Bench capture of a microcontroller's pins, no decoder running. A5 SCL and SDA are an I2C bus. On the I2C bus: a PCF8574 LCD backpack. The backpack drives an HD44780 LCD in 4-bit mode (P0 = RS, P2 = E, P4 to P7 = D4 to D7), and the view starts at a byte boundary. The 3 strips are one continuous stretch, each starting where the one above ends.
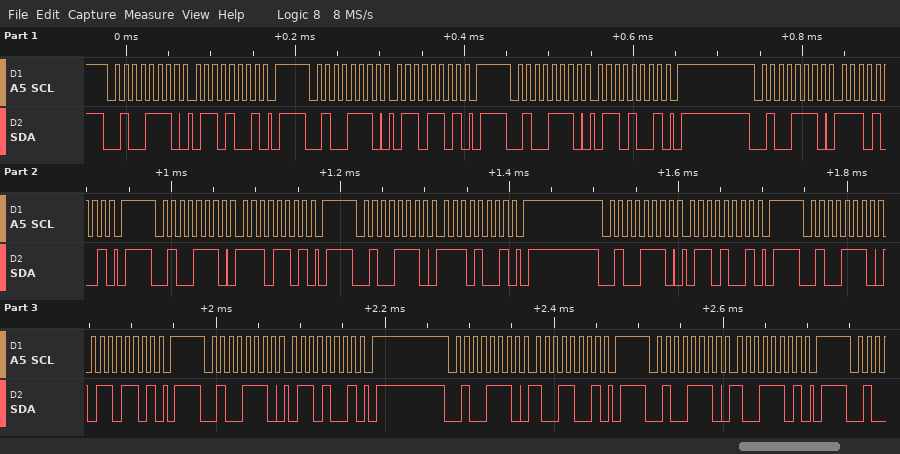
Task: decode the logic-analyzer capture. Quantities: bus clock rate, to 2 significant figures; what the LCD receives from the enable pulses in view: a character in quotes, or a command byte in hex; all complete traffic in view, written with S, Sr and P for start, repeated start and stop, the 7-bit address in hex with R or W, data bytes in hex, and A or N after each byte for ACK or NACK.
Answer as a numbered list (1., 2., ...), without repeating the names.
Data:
1. 100 kHz
2. 'n'
3. S 27W A 69 A P S 27W A 6D A P S 27W A 69 A P S 27W A E9 A P S 27W A ED A P S 27W A E9 A P S 27W A 69 A P S 27W A 6D A P S 27W A 69 A P S 27W A 99 A P S 27W A 9D A P
